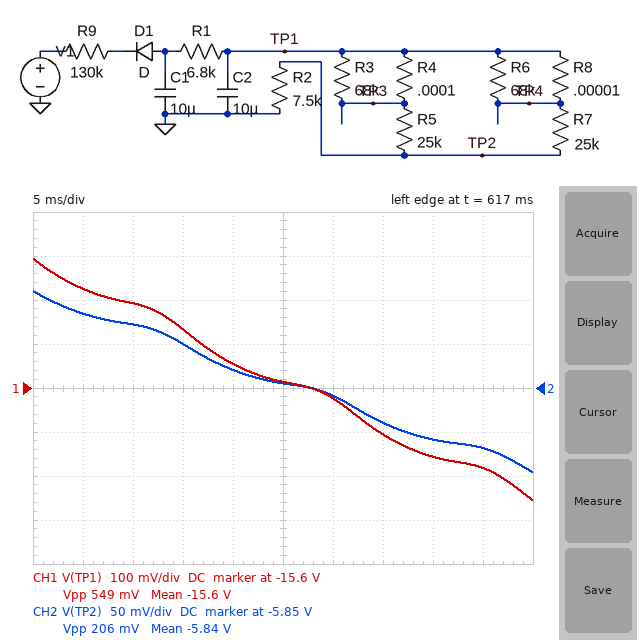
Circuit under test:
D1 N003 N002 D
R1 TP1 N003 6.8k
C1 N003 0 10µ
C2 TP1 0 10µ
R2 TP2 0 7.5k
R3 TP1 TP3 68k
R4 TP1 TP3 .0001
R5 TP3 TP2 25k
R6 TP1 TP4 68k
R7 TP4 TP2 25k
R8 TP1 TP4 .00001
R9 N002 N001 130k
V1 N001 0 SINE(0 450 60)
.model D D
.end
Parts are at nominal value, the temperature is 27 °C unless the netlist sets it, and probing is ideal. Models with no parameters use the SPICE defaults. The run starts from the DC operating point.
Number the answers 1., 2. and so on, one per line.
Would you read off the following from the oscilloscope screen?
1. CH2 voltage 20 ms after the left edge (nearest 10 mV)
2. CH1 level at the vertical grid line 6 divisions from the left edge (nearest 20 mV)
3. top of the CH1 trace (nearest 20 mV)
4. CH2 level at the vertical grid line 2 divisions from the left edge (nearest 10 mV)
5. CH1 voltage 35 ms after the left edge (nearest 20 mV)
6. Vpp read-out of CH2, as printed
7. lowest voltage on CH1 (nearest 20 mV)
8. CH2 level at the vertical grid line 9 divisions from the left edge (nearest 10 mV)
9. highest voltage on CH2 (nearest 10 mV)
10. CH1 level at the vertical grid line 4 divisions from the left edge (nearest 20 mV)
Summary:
1. -5.83 V
2. -15.62 V
3. -15.30 V
4. -5.78 V
5. -15.70 V
6. 206 mV
7. -15.86 V
8. -5.92 V
9. -5.74 V
10. -15.54 V
